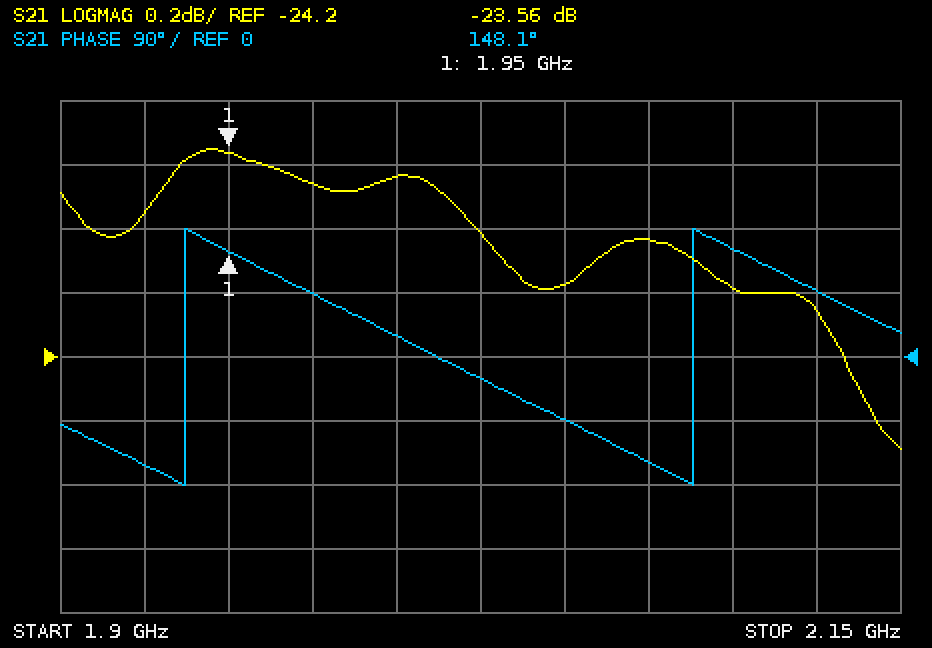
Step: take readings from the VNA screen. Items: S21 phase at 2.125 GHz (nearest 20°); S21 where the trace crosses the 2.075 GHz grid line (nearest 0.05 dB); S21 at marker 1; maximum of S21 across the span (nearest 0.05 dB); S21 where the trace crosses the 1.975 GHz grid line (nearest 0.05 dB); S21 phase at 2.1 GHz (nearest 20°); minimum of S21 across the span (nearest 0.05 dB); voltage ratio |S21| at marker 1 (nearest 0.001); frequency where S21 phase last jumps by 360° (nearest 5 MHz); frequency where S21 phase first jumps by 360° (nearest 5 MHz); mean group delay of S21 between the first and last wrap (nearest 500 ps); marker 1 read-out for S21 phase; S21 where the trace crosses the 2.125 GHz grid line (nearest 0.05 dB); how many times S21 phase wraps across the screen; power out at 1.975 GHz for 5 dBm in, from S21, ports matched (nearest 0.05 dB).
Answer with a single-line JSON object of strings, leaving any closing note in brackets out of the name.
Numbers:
{"S21 phase at 2.125 GHz": "100°", "S21 where the trace crosses the 2.075 GHz grid line": "-23.85 dB", "S21 at marker 1": "-23.56 dB", "maximum of S21 across the span": "-23.55 dB", "S21 where the trace crosses the 1.975 GHz grid line": "-23.65 dB", "S21 phase at 2.1 GHz": "160°", "minimum of S21 across the span": "-24.50 dB", "voltage ratio |S21| at marker 1": "0.066", "frequency where S21 phase last jumps by 360°": "2.090 GHz", "frequency where S21 phase first jumps by 360°": "1.935 GHz", "mean group delay of S21 between the first and last wrap": "6.5 ns", "marker 1 read-out for S21 phase": "148.1°", "S21 where the trace crosses the 2.125 GHz grid line": "-24.05 dB", "how many times S21 phase wraps across the screen": "2", "power out at 1.975 GHz for 5 dBm in, from S21, ports matched": "-18.65 dBm"}
